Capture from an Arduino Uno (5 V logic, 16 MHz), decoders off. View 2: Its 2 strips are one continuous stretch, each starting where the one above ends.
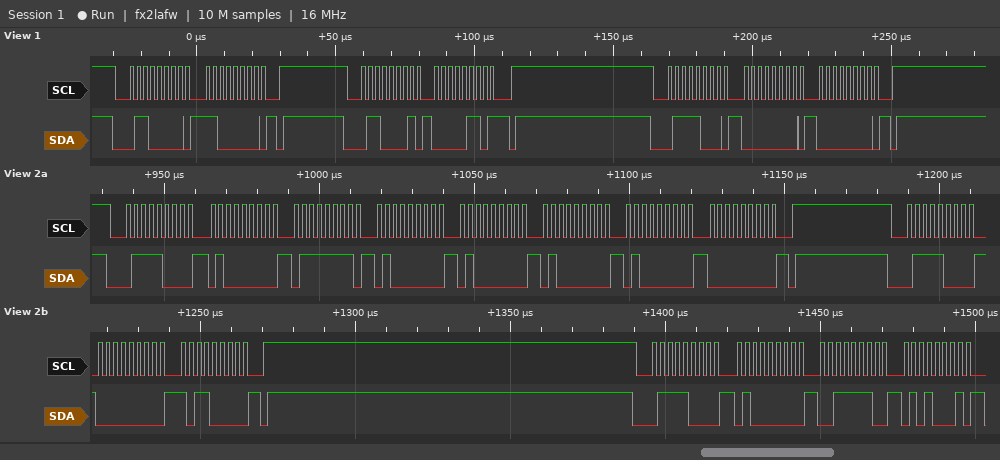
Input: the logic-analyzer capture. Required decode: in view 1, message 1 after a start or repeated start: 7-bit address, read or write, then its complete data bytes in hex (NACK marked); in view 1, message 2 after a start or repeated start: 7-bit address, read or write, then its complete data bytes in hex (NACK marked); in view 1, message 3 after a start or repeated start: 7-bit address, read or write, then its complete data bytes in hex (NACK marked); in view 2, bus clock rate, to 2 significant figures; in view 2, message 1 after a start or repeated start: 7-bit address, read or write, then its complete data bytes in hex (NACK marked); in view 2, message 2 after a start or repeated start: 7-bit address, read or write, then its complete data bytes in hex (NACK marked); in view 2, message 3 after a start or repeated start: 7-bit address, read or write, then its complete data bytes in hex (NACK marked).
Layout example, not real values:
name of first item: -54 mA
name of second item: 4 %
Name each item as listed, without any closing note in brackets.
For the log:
in view 1, message 1 after a start or repeated start: 7-bit address, read or write, then its complete data bytes in hex: 0x30 write: C0
in view 1, message 2 after a start or repeated start: 7-bit address, read or write, then its complete data bytes in hex: 0x30 read: 06 NACK
in view 1, message 3 after a start or repeated start: 7-bit address, read or write, then its complete data bytes in hex: 0x3C write: 00 00
in view 2, bus clock rate, to 2 significant figures: 400 kHz
in view 2, message 1 after a start or repeated start: 7-bit address, read or write, then its complete data bytes in hex: 0x3C write: 40 7F 40 40 40 40 00
in view 2, message 2 after a start or repeated start: 7-bit address, read or write, then its complete data bytes in hex: 0x3C write: 00 B0
in view 2, message 3 after a start or repeated start: 7-bit address, read or write, then its complete data bytes in hex: 0x3C write: 40 3E 51
